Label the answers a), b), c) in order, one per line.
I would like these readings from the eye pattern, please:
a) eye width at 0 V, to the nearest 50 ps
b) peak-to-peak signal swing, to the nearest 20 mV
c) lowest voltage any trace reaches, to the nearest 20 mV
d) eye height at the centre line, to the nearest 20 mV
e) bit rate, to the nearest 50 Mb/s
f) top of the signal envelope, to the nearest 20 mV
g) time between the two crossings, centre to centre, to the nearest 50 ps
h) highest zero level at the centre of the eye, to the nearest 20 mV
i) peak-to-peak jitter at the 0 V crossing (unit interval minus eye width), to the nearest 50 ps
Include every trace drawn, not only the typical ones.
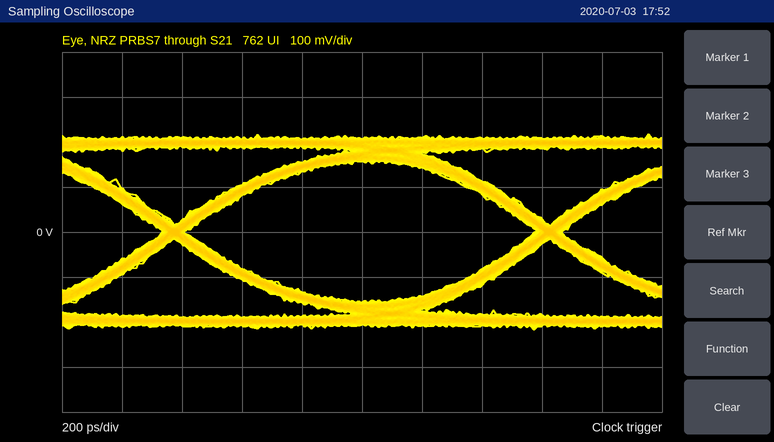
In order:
a) 1.15 ns
b) 440 mV
c) -220 mV
d) 320 mV
e) 800 Mb/s
f) 220 mV
g) 1.25 ns
h) -160 mV
i) 100 ps
